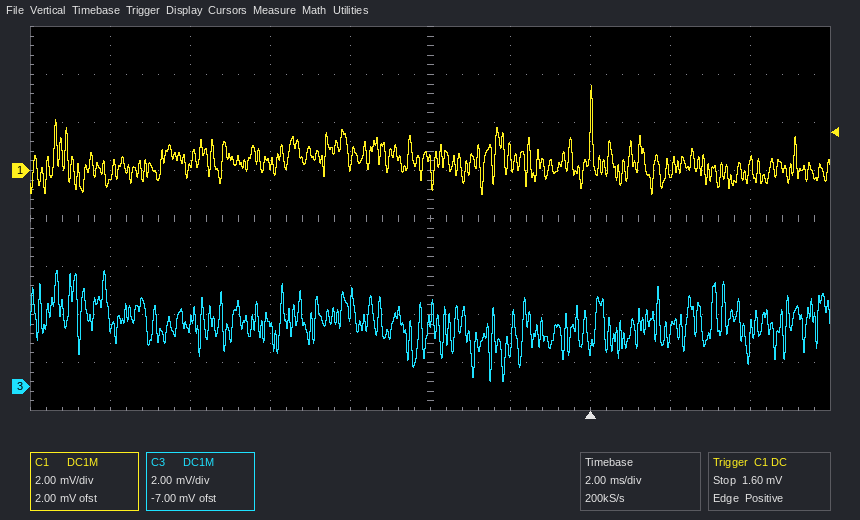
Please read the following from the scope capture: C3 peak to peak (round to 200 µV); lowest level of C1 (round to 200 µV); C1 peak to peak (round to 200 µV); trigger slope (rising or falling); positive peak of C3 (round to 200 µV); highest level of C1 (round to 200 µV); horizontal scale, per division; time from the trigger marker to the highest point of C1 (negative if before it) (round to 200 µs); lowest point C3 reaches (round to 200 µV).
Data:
4.6 mV
-1.0 mV
4.6 mV
rising
4.8 mV
3.6 mV
2 ms
0.0 ms
200 µV
